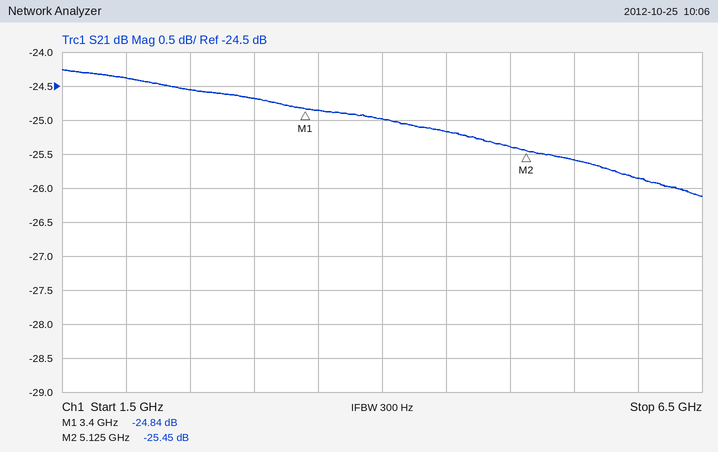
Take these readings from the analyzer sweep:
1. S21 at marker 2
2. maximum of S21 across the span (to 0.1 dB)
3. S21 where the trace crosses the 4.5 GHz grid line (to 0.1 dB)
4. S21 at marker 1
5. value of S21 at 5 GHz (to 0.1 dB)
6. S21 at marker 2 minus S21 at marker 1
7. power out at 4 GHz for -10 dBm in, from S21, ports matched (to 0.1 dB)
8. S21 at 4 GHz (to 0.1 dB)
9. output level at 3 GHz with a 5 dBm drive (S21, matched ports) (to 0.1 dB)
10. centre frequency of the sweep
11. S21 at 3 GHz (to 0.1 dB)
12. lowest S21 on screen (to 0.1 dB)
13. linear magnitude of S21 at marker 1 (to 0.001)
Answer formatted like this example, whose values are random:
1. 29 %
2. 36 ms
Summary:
1. -25.45 dB
2. -24.3 dB
3. -25.2 dB
4. -24.84 dB
5. -25.4 dB
6. -0.61 dB
7. -35.0 dBm
8. -25.0 dB
9. -19.7 dBm
10. 4 GHz
11. -24.7 dB
12. -26.1 dB
13. 0.057
